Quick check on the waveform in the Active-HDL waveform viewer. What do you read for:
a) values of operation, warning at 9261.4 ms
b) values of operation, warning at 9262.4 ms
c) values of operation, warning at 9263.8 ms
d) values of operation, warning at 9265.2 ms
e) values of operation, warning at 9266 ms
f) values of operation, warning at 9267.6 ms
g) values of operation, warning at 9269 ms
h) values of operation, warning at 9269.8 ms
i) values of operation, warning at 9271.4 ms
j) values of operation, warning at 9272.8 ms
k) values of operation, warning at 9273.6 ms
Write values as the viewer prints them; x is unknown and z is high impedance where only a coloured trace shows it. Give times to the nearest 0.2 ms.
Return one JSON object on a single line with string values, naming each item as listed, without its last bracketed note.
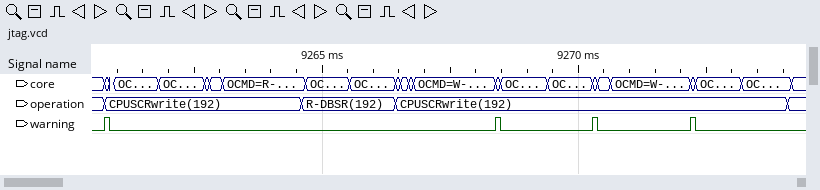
{"values of operation, warning at 9261.4 ms": "operation=CPUSCRwrite(192), warning=0", "values of operation, warning at 9262.4 ms": "operation=CPUSCRwrite(192), warning=0", "values of operation, warning at 9263.8 ms": "operation=CPUSCRwrite(192), warning=0", "values of operation, warning at 9265.2 ms": "operation=R-DBSR(192), warning=0", "values of operation, warning at 9266 ms": "operation=R-DBSR(192), warning=0", "values of operation, warning at 9267.6 ms": "operation=CPUSCRwrite(192), warning=0", "values of operation, warning at 9269 ms": "operation=CPUSCRwrite(192), warning=0", "values of operation, warning at 9269.8 ms": "operation=CPUSCRwrite(192), warning=0", "values of operation, warning at 9271.4 ms": "operation=CPUSCRwrite(192), warning=0", "values of operation, warning at 9272.8 ms": "operation=CPUSCRwrite(192), warning=0", "values of operation, warning at 9273.6 ms": "operation=CPUSCRwrite(192), warning=0"}
